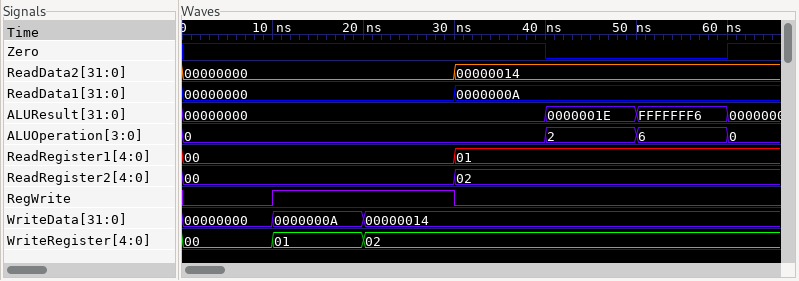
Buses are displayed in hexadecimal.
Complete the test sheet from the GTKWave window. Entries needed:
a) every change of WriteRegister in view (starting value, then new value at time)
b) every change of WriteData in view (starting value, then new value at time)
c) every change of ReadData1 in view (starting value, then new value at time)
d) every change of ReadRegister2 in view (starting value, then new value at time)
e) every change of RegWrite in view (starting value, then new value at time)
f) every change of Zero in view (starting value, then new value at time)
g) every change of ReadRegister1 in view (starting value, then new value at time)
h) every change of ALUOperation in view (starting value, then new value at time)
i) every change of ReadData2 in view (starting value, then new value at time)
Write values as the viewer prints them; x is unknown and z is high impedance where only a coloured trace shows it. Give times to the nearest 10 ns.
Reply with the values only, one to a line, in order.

00, 01 at 10 ns, 02 at 20 ns
00000000, 0000000A at 10 ns, 00000014 at 20 ns
00000000, 0000000A at 30 ns
00, 02 at 30 ns
0, 1 at 10 ns, 0 at 30 ns
1, 0 at 40 ns, 1 at 60 ns
00, 01 at 30 ns
0, 2 at 40 ns, 6 at 50 ns, 0 at 60 ns
00000000, 00000014 at 30 ns
